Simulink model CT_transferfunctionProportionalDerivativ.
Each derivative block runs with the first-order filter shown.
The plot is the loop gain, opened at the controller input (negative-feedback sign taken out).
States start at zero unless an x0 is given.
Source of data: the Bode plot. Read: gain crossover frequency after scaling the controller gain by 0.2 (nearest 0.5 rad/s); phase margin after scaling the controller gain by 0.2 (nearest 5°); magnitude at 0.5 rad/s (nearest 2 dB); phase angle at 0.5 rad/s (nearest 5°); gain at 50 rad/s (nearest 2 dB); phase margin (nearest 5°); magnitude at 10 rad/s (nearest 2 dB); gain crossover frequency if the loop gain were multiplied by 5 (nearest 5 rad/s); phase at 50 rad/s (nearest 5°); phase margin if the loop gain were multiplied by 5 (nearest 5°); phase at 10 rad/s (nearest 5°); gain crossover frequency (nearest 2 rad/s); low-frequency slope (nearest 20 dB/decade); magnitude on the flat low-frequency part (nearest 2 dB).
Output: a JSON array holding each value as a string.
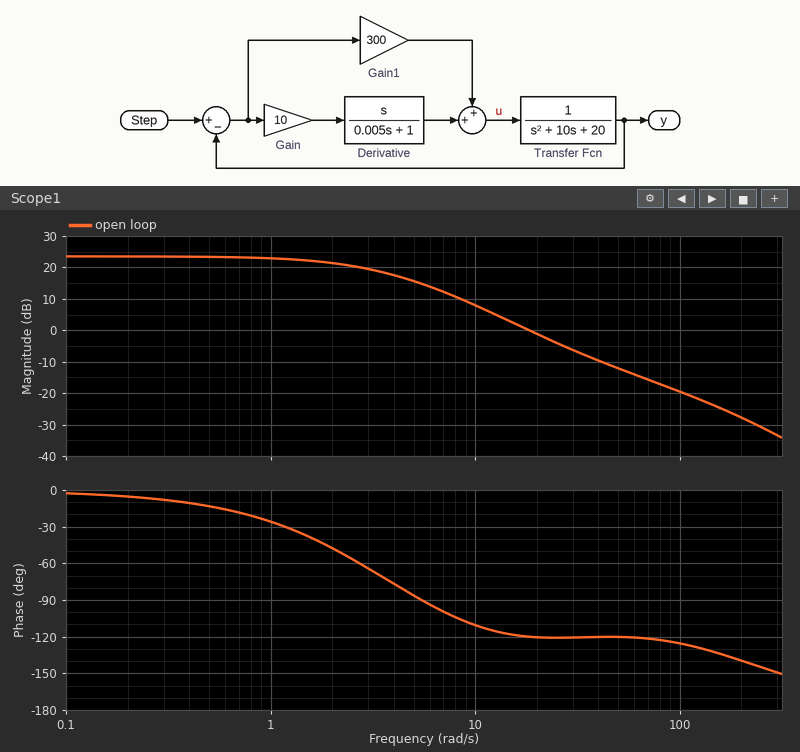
["6.0 rad/s", "85°", "24 dB", "-15°", "-12 dB", "60°", "8 dB", "60 rad/s", "-120°", "60°", "-110°", "18 rad/s", "0 dB/decade", "24 dB"]
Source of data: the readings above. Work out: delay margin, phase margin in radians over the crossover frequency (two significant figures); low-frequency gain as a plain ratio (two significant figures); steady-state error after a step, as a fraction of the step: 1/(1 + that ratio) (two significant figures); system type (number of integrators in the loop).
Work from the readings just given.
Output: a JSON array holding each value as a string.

["0.058 s", "16", "0.059", "0"]
